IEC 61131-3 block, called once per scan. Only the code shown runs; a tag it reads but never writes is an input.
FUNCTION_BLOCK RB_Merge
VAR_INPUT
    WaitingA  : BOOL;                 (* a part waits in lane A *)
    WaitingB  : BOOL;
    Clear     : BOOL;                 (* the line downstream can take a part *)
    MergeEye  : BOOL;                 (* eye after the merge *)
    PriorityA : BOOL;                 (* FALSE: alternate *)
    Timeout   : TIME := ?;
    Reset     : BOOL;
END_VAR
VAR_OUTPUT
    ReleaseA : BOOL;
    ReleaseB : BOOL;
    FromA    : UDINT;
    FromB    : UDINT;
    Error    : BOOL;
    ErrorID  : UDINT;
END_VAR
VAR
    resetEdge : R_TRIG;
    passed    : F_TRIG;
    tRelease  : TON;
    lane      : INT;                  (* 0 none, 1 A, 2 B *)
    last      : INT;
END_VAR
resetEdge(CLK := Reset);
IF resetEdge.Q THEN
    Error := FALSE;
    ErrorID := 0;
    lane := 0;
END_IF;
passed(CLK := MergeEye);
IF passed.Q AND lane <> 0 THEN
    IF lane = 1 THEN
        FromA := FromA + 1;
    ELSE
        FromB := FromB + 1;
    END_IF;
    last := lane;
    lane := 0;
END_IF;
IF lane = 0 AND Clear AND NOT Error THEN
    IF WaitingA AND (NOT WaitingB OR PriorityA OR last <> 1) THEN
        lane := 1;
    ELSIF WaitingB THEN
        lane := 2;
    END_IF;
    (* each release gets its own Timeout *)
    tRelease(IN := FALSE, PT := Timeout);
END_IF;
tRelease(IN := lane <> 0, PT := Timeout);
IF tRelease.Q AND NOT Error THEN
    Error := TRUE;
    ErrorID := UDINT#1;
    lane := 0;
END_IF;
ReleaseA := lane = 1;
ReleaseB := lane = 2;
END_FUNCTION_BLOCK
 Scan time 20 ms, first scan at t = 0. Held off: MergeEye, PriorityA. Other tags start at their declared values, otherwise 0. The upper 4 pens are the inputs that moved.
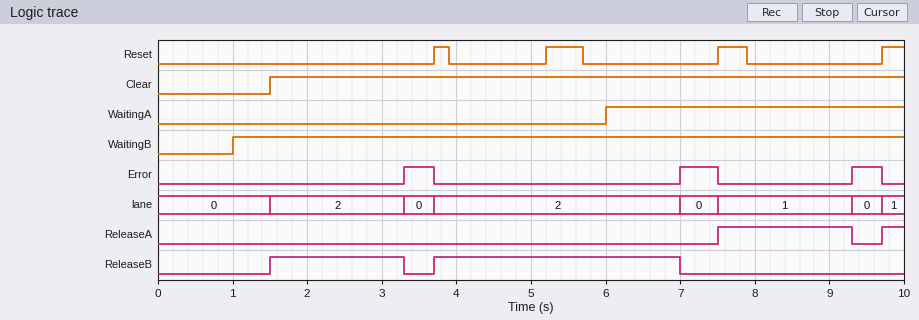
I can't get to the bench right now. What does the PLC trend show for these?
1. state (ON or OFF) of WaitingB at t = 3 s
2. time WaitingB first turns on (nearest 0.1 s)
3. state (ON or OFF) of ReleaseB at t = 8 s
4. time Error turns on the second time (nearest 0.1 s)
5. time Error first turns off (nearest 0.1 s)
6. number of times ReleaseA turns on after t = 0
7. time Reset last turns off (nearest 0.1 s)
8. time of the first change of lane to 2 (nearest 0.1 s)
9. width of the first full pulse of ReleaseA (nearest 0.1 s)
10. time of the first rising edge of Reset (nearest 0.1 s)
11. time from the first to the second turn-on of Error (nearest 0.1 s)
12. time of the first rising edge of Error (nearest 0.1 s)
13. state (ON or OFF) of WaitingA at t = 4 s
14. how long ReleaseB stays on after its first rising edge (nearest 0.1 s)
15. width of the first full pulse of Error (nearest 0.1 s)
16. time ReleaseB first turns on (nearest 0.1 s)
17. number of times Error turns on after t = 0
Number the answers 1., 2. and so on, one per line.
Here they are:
1. ON
2. 1.0 s
3. OFF
4. 7.0 s
5. 3.7 s
6. 2
7. 7.9 s
8. 1.5 s
9. 1.8 s
10. 3.7 s
11. 3.7 s
12. 3.3 s
13. OFF
14. 1.8 s
15. 0.4 s
16. 1.5 s
17. 3
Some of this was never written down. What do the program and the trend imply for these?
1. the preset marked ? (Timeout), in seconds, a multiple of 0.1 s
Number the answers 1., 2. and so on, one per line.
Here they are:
1. 1.8 s
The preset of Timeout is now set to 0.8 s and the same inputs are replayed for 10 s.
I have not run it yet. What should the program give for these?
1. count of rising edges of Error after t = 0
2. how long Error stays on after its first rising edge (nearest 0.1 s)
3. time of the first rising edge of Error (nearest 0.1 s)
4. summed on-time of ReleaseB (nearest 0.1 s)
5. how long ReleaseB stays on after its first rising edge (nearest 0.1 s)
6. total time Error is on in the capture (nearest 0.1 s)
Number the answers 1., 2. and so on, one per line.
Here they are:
1. 4
2. 1.4 s
3. 2.3 s
4. 2.4 s
5. 0.8 s
6. 5.0 s
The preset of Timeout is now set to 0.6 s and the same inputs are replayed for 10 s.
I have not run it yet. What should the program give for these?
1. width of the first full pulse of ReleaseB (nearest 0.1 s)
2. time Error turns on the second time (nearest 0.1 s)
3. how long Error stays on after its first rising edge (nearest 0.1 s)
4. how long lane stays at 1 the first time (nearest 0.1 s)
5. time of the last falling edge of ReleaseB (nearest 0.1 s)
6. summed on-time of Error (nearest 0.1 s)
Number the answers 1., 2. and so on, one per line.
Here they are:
1. 0.6 s
2. 4.3 s
3. 1.6 s
4. 0.6 s
5. 5.8 s
6. 5.8 s
